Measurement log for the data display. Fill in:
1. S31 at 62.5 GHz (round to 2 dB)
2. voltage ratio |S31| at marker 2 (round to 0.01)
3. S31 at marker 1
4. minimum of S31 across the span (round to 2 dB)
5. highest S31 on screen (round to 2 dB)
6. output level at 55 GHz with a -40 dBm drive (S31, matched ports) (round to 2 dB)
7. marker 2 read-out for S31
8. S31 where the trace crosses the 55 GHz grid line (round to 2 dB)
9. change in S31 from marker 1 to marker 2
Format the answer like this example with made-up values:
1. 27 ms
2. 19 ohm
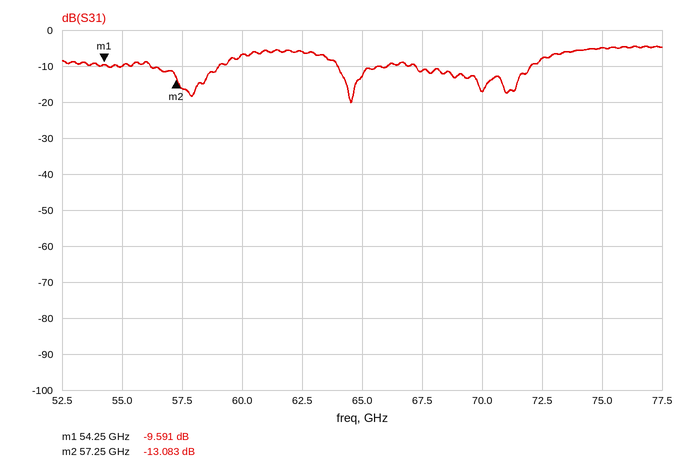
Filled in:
1. -6 dB
2. 0.22
3. -9.591 dB
4. -20 dB
5. -4 dB
6. -50 dBm
7. -13.083 dB
8. -10 dB
9. -3.492 dB
